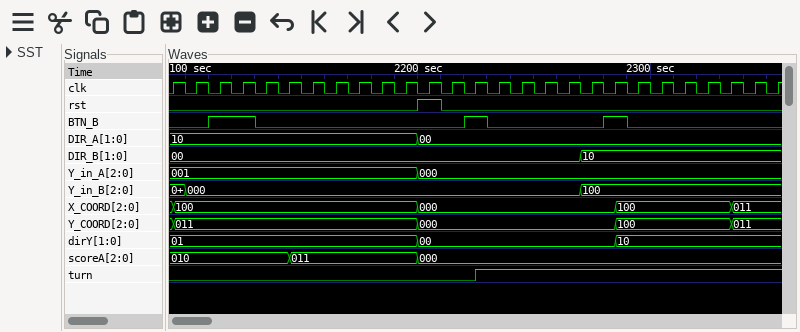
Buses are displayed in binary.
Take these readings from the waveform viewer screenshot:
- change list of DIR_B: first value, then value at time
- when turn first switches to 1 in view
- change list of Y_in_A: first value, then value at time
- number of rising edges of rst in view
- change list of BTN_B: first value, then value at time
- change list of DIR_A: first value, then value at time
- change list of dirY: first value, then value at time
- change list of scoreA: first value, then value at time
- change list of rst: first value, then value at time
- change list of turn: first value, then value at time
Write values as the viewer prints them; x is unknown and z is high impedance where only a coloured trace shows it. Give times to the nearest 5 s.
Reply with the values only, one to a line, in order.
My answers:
00, 10 at 2270 s
2225 s
001, 000 at 2200 s
1
0, 1 at 2110 s, 0 at 2130 s, 1 at 2220 s, 0 at 2230 s, 1 at 2280 s, 0 at 2290 s
10, 00 at 2200 s
01, 00 at 2200 s, 10 at 2285 s
010, 011 at 2145 s, 000 at 2200 s
0, 1 at 2200 s, 0 at 2210 s
0, 1 at 2225 s
